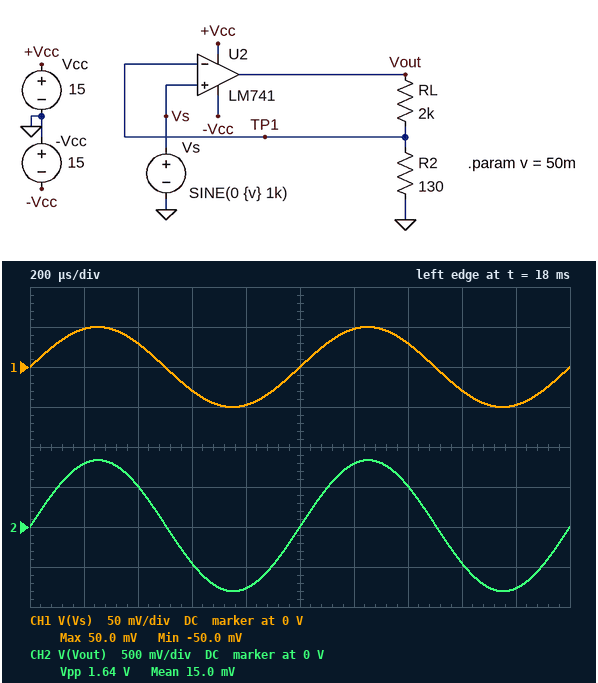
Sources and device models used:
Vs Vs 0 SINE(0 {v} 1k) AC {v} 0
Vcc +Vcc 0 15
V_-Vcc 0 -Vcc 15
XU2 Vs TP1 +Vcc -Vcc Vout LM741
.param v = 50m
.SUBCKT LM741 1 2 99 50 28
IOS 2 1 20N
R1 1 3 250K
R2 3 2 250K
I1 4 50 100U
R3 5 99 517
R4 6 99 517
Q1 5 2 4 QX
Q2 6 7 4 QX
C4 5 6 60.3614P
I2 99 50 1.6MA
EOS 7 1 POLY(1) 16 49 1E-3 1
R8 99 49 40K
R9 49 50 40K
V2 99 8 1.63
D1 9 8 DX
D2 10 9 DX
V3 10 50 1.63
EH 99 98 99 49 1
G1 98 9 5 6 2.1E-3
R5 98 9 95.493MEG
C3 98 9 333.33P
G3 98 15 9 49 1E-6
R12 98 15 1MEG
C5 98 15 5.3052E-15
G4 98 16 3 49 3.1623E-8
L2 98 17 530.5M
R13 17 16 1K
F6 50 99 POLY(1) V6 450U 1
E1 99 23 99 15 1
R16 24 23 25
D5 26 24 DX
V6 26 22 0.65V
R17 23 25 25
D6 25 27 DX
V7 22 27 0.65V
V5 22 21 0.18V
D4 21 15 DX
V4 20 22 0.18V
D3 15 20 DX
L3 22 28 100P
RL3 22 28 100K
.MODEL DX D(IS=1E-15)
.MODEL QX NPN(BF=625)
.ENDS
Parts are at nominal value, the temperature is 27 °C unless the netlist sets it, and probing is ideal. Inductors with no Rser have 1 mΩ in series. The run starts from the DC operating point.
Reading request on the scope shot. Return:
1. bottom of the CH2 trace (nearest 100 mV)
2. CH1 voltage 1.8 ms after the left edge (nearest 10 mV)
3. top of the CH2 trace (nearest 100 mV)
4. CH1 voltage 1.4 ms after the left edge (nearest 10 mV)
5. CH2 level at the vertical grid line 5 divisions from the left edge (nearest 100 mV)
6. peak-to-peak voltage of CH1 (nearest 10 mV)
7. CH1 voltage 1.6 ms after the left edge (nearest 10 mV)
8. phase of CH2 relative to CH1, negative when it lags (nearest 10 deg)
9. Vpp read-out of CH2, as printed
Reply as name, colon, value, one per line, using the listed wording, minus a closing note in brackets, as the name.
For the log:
bottom of the CH2 trace: -800 mV
CH1 voltage 1.8 ms after the left edge: -50 mV
top of the CH2 trace: 800 mV
CH1 voltage 1.4 ms after the left edge: 30 mV
CH2 level at the vertical grid line 5 divisions from the left edge: 0 V
peak-to-peak voltage of CH1: 100 mV
CH1 voltage 1.6 ms after the left edge: -30 mV
phase of CH2 relative to CH1, negative when it lags: 0 deg
Vpp read-out of CH2, as printed: 1.64 V
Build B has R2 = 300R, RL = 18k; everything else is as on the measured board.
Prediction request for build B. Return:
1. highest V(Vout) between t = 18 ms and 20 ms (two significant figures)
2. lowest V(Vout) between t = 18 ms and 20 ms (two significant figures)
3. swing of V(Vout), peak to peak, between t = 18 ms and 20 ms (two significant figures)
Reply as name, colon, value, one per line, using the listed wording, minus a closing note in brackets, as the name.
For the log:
highest V(Vout) between t = 18 ms and 20 ms: 3.1 V
lowest V(Vout) between t = 18 ms and 20 ms: -3.0 V
swing of V(Vout), peak to peak, between t = 18 ms and 20 ms: 6.1 V
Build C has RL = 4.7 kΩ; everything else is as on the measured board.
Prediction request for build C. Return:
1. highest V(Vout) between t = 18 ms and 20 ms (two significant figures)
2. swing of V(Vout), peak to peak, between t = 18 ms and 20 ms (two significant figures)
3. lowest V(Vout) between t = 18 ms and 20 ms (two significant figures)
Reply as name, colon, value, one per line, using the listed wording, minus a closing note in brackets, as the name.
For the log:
highest V(Vout) between t = 18 ms and 20 ms: 1.9 V
swing of V(Vout), peak to peak, between t = 18 ms and 20 ms: 3.7 V
lowest V(Vout) between t = 18 ms and 20 ms: -1.8 V
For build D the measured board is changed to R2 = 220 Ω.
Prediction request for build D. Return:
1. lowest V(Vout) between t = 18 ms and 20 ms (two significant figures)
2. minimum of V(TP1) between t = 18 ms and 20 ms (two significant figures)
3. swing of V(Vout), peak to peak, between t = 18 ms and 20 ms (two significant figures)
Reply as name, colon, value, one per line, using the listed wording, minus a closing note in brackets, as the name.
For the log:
lowest V(Vout) between t = 18 ms and 20 ms: -490 mV
minimum of V(TP1) between t = 18 ms and 20 ms: -49 mV
swing of V(Vout), peak to peak, between t = 18 ms and 20 ms: 1.0 V
